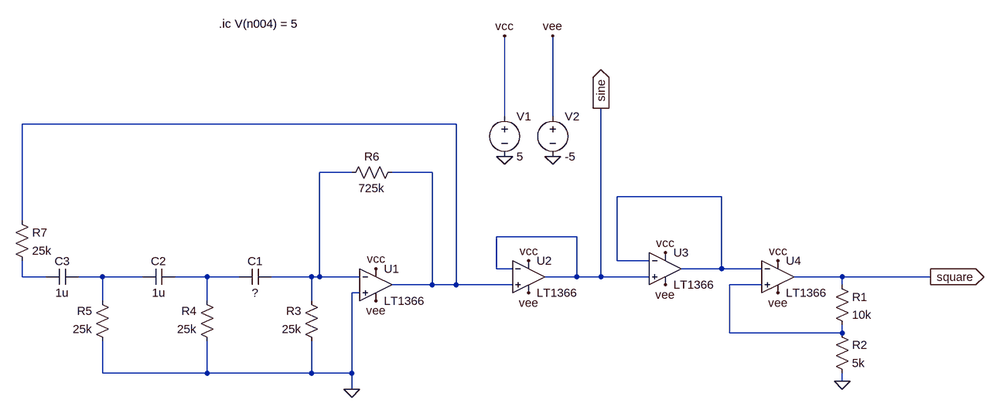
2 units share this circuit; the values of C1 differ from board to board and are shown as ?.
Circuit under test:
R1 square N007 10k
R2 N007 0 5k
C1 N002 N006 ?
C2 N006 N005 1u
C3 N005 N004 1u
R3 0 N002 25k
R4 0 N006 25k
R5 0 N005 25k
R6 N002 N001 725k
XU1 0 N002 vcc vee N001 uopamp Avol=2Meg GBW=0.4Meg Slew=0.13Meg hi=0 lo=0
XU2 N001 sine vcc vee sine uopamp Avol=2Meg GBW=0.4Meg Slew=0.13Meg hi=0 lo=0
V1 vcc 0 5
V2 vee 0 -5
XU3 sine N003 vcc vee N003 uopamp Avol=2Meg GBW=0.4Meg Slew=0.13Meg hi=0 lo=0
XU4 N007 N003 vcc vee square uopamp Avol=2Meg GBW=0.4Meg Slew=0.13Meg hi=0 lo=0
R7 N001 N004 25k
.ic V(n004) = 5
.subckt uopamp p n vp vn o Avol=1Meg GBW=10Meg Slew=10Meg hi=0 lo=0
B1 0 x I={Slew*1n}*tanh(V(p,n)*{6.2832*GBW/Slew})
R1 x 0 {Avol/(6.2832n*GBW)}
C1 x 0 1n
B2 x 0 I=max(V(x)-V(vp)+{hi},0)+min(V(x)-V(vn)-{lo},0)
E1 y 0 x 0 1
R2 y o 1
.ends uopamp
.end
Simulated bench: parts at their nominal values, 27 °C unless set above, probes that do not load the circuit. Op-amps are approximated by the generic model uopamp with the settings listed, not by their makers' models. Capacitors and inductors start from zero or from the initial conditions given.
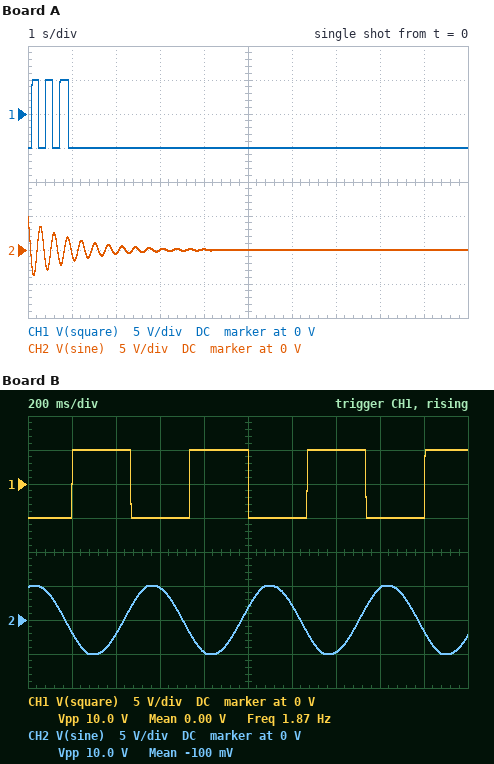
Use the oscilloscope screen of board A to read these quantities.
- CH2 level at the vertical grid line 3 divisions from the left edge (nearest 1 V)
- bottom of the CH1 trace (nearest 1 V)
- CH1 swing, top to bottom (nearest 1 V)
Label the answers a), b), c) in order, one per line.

a) 0 V
b) -5 V
c) 10 V
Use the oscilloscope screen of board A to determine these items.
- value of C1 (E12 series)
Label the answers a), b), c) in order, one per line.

a) 560 nF
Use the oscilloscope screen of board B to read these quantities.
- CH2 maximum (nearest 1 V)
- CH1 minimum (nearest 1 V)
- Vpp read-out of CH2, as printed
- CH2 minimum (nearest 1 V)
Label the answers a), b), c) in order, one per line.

a) 5 V
b) -5 V
c) 10.0 V
d) -5 V
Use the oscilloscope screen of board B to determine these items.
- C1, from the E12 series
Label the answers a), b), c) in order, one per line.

a) 2.7 µF
